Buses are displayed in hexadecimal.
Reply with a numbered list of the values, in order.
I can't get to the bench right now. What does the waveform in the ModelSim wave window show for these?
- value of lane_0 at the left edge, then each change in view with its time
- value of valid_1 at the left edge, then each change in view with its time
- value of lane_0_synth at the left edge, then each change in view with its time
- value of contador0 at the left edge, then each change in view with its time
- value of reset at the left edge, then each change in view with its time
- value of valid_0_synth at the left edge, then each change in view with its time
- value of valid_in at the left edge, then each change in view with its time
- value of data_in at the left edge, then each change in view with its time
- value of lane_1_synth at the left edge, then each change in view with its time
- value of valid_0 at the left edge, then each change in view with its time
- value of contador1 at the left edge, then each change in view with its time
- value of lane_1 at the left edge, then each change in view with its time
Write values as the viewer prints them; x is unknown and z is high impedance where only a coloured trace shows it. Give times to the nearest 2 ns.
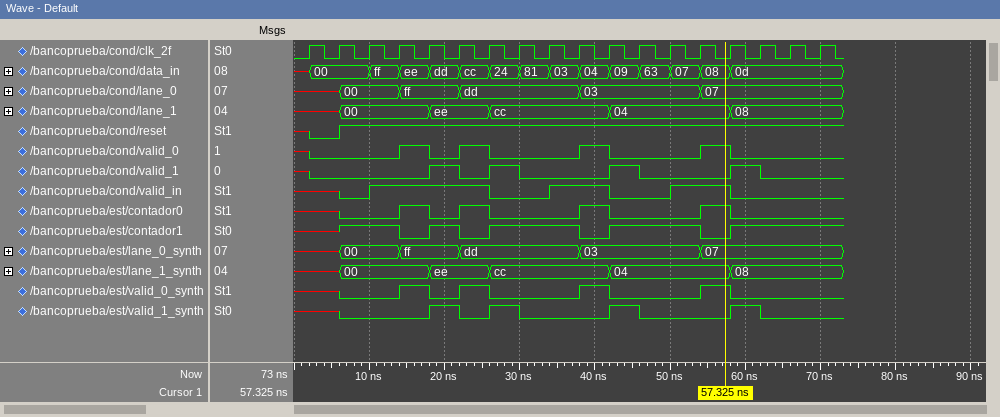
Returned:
1. x, 00 at 6 ns, ff at 14 ns, dd at 22 ns, 03 at 38 ns, 07 at 54 ns
2. x, 0 at 2 ns, 1 at 18 ns, 0 at 22 ns, 1 at 26 ns, 0 at 30 ns, 1 at 42 ns, 0 at 46 ns, 1 at 58 ns, 0 at 62 ns
3. x, 00 at 6 ns, ff at 14 ns, dd at 22 ns, 03 at 38 ns, 07 at 54 ns
4. x, 0 at 6 ns, 1 at 14 ns, 0 at 18 ns, 1 at 22 ns, 0 at 26 ns, 1 at 38 ns, 0 at 42 ns, 1 at 54 ns, 0 at 58 ns
5. x, 0 at 2 ns, 1 at 6 ns
6. x, 0 at 6 ns, 1 at 14 ns, 0 at 18 ns, 1 at 22 ns, 0 at 26 ns, 1 at 38 ns, 0 at 42 ns, 1 at 54 ns, 0 at 58 ns
7. x, 0 at 6 ns, 1 at 10 ns, 0 at 26 ns, 1 at 34 ns, 0 at 42 ns, 1 at 50 ns, 0 at 58 ns
8. x, 00 at 2 ns, ff at 10 ns, ee at 14 ns, dd at 18 ns, cc at 22 ns, 24 at 26 ns, 81 at 30 ns, 03 at 34 ns, 04 at 38 ns, 09 at 42 ns, 63 at 46 ns, 07 at 50 ns, 08 at 54 ns, 0d at 58 ns
9. x, 00 at 6 ns, ee at 18 ns, cc at 26 ns, 04 at 42 ns, 08 at 58 ns
10. x, 0 at 2 ns, 1 at 14 ns, 0 at 18 ns, 1 at 22 ns, 0 at 26 ns, 1 at 38 ns, 0 at 42 ns, 1 at 54 ns, 0 at 58 ns
11. x, 1 at 6 ns, 0 at 14 ns, 1 at 18 ns, 0 at 22 ns, 1 at 26 ns, 0 at 38 ns, 1 at 42 ns, 0 at 54 ns, 1 at 58 ns
12. x, 00 at 6 ns, ee at 18 ns, cc at 26 ns, 04 at 42 ns, 08 at 58 ns
